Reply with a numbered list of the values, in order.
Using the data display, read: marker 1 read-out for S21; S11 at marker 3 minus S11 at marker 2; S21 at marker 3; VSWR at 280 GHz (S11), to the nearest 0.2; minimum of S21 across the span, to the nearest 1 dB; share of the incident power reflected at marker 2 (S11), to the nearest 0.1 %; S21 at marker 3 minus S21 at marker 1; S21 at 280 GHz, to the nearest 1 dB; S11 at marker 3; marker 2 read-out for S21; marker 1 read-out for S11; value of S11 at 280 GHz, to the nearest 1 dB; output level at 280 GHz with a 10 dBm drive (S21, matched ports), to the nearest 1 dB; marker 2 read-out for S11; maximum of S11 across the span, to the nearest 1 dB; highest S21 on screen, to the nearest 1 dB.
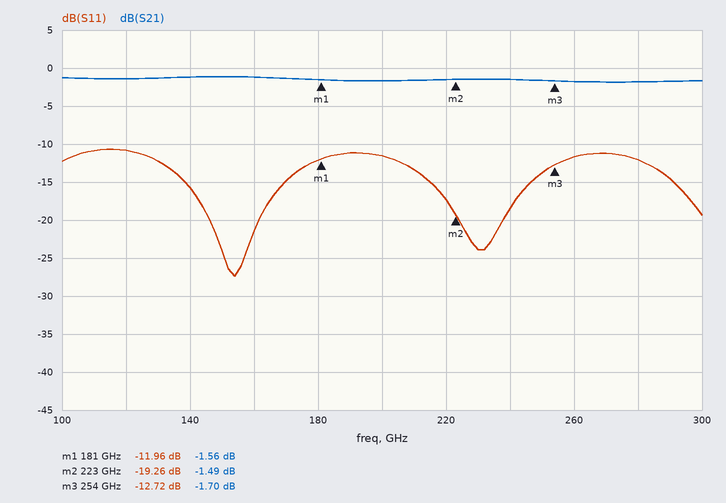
1. -1.56 dB
2. 6.54 dB
3. -1.70 dB
4. 1.6
5. -2 dB
6. 1.2 %
7. -0.14 dB
8. -2 dB
9. -12.72 dB
10. -1.49 dB
11. -11.96 dB
12. -12 dB
13. 8 dBm
14. -19.26 dB
15. -11 dB
16. -1 dB
